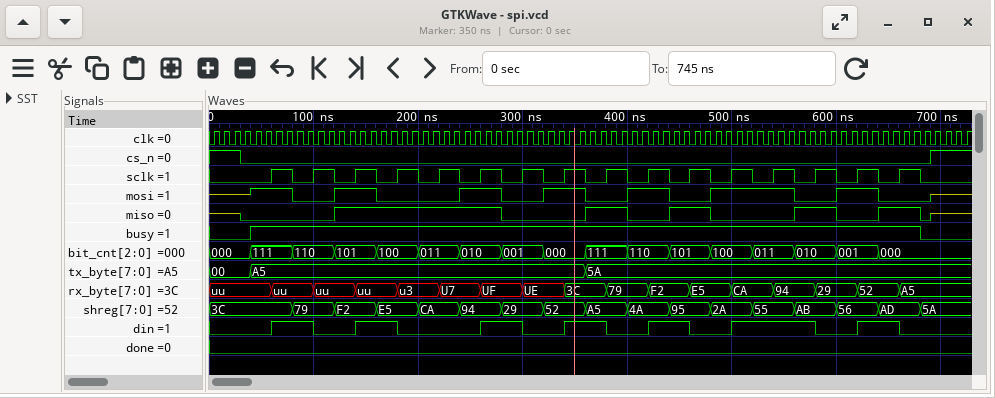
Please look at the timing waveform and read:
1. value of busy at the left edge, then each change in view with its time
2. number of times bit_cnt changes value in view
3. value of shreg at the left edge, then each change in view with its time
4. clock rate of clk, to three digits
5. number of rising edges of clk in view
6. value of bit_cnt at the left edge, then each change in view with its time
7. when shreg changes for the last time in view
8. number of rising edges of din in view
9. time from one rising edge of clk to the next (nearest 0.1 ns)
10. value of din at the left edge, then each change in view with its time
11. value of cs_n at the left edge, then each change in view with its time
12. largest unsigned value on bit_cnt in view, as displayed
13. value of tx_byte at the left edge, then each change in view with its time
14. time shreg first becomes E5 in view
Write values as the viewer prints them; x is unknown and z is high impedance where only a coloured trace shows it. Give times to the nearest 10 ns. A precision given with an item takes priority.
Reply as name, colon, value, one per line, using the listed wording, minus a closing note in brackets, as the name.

value of busy at the left edge, then each change in view with its time: 0, 1 at 40 ns, 0 at 680 ns
number of times bit_cnt changes value in view: 16
value of shreg at the left edge, then each change in view with its time: 3C, 79 at 80 ns, F2 at 120 ns, E5 at 160 ns, CA at 200 ns, 94 at 240 ns, 29 at 280 ns, 52 at 320 ns, A5 at 360 ns, 4A at 400 ns, 95 at 440 ns, 2A at 480 ns, 55 at 520 ns, AB at 560 ns, 56 at 600 ns, AD at 640 ns, 5A at 680 ns
clock rate of clk, to three digits: 100 MHz
number of rising edges of clk in view: 73
value of bit_cnt at the left edge, then each change in view with its time: 000, 111 at 40 ns, 110 at 80 ns, 101 at 120 ns, 100 at 160 ns, 011 at 200 ns, 010 at 240 ns, 001 at 280 ns, 000 at 320 ns, 111 at 360 ns, 110 at 400 ns, 101 at 440 ns, 100 at 480 ns, 011 at 520 ns, 010 at 560 ns, 001 at 600 ns, 000 at 640 ns
when shreg changes for the last time in view: 680 ns
number of rising edges of din in view: 7
time from one rising edge of clk to the next: 10 ns
value of din at the left edge, then each change in view with its time: 0, 1 at 60 ns, 0 at 100 ns, 1 at 140 ns, 0 at 180 ns, 1 at 260 ns, 0 at 300 ns, 1 at 340 ns, 0 at 380 ns, 1 at 420 ns, 0 at 460 ns, 1 at 500 ns, 0 at 580 ns, 1 at 620 ns, 0 at 660 ns
value of cs_n at the left edge, then each change in view with its time: 1, 0 at 30 ns, 1 at 690 ns
largest unsigned value on bit_cnt in view, as displayed: 111
value of tx_byte at the left edge, then each change in view with its time: 00, A5 at 40 ns, 5A at 360 ns
time shreg first becomes E5 in view: 160 ns
